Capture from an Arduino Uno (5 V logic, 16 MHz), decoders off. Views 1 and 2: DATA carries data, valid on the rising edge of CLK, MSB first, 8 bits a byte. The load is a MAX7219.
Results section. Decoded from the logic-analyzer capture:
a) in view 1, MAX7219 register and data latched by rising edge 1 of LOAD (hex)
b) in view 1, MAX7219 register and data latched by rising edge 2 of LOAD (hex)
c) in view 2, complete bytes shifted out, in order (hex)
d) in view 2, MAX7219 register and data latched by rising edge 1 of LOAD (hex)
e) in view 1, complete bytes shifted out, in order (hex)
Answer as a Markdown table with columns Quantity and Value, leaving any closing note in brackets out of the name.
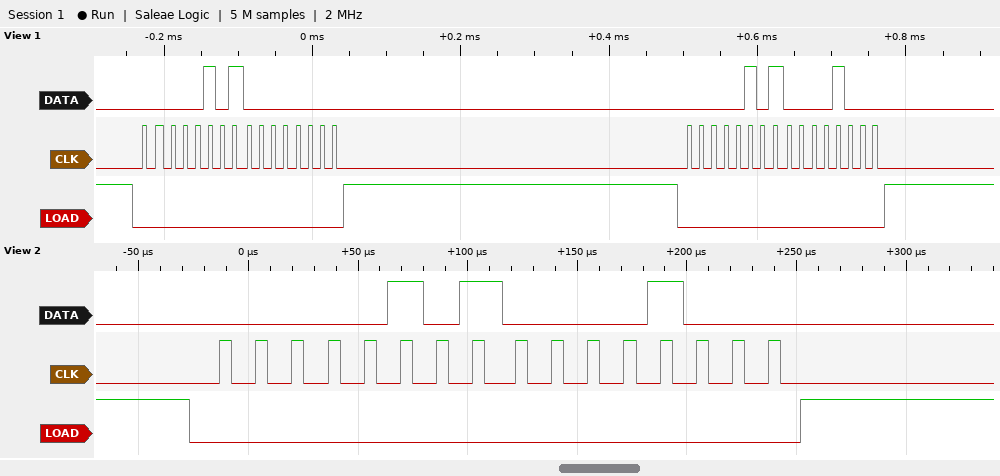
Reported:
| Quantity | Value |
|---|---|
| in view 1, MAX7219 register and data latched by rising edge 1 of LOAD | register 0x5, data 0x00 |
| in view 1, MAX7219 register and data latched by rising edge 2 of LOAD | register 0x5, data 0x08 |
| in view 2, complete bytes shifted out, in order | 05 08 |
| in view 2, MAX7219 register and data latched by rising edge 1 of LOAD | register 0x5, data 0x08 |
| in view 1, complete bytes shifted out, in order | 0x05 0x00 0x05 0x08 |
